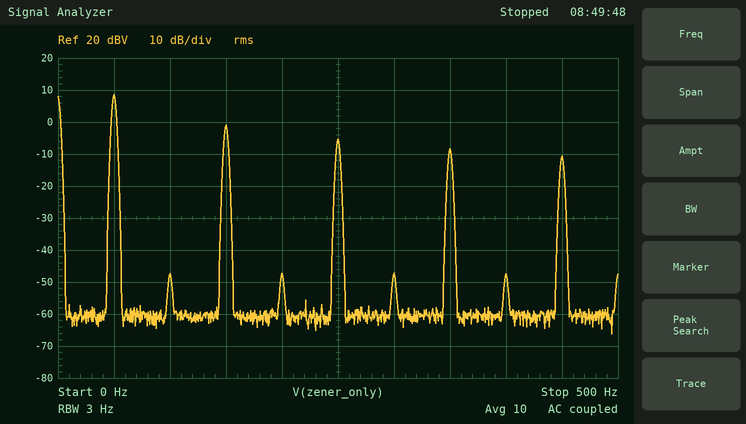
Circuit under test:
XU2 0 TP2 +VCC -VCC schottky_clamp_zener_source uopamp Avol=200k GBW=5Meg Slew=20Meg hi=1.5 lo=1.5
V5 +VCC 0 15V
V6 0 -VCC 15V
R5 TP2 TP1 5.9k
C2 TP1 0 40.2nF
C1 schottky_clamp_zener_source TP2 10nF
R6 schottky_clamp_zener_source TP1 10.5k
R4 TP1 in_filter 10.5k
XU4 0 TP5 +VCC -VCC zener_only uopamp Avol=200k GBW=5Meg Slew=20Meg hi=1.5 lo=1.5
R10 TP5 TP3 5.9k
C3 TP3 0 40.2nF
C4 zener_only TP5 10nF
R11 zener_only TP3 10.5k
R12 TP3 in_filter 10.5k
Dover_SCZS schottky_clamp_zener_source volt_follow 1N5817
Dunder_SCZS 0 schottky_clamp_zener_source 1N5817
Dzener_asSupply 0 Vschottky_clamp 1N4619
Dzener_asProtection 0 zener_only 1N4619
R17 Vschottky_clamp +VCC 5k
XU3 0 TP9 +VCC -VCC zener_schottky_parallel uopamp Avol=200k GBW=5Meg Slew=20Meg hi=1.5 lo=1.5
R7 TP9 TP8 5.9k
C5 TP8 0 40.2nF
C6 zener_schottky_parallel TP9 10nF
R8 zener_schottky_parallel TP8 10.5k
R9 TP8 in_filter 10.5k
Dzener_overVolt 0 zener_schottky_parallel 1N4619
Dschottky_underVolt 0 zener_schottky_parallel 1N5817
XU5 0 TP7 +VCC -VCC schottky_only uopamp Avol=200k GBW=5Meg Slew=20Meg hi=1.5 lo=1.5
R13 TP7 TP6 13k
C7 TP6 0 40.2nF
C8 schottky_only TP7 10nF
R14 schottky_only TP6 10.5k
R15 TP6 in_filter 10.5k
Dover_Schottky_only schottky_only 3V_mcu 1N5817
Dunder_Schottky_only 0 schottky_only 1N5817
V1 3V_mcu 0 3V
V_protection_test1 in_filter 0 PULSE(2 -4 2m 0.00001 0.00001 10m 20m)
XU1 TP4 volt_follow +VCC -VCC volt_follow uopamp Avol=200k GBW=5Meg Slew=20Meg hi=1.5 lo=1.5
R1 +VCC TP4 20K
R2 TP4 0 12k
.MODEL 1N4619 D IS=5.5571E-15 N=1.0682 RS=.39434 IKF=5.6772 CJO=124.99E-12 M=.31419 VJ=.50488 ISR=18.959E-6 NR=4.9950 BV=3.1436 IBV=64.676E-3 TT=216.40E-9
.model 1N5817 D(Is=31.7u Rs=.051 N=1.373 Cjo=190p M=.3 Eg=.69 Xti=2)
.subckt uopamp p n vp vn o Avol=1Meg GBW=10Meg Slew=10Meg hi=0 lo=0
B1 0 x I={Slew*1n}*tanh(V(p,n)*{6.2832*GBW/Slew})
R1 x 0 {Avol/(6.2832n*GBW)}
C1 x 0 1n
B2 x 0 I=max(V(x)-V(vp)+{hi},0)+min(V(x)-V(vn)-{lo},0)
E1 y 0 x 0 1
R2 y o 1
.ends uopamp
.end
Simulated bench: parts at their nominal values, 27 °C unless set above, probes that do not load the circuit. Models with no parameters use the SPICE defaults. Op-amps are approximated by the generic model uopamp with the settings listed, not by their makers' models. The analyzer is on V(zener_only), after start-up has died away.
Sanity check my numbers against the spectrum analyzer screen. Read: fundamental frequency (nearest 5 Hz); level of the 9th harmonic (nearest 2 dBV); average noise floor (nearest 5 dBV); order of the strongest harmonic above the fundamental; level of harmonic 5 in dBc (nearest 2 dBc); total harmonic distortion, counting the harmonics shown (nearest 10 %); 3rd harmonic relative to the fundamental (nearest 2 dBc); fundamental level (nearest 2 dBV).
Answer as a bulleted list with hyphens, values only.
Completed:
- 50 Hz
- -10 dBV
- -60 dBV
- 3
- -14 dBc
- 40 %
- -10 dBc
- 8 dBV
